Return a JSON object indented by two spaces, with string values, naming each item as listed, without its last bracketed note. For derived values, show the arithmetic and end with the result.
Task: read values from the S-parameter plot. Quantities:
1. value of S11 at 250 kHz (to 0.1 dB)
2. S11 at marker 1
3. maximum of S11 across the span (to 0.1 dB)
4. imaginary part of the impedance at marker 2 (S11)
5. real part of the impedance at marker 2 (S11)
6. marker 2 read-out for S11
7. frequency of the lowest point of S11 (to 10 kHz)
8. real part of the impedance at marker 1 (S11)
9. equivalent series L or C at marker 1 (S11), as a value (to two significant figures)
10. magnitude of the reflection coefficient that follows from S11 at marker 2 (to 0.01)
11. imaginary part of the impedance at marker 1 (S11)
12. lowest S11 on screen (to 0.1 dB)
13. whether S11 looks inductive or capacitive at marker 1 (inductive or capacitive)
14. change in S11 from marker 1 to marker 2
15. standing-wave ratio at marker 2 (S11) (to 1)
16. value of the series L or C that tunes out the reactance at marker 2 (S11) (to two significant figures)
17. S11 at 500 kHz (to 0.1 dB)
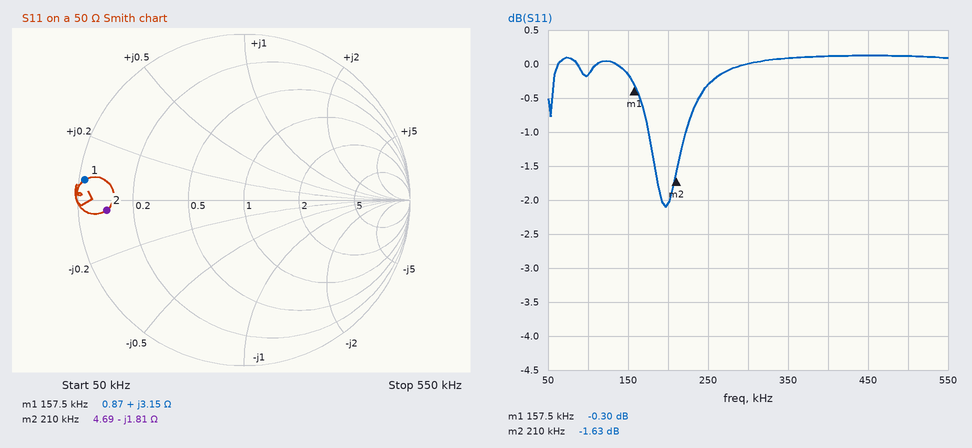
{
  "value of S11 at 250 kHz": "-0.3 dB",
  "S11 at marker 1": "-0.30 dB",
  "maximum of S11 across the span": "0.1 dB",
  "imaginary part of the impedance at marker 2": "-1.81 Ω",
  "real part of the impedance at marker 2": "4.69 Ω",
  "marker 2 read-out for S11": "-1.63 dB",
  "frequency of the lowest point of S11": "200 kHz",
  "real part of the impedance at marker 1": "0.87 Ω",
  "equivalent series L or C at marker 1 (S11), as a value": "L = 3.15 Ω/(2π × 157.5 kHz) ≈ 3.2 µH",
  "magnitude of the reflection coefficient that follows from S11 at marker 2": "10^(-1.63/20) ≈ 0.83",
  "imaginary part of the impedance at marker 1": "+3.15 Ω",
  "lowest S11 on screen": "-2.1 dB",
  "whether S11 looks inductive or capacitive at marker 1": "inductive",
  "change in S11 from marker 1 to marker 2": "-1.63 − (-0.3) = -1.33 dB",
  "standing-wave ratio at marker 2 (S11)": "11",
  "value of the series L or C that tunes out the reactance at marker 2 (S11)": "L = 1.81 Ω/(2π × 210 kHz) ≈ 1.4 µH",
  "S11 at 500 kHz": "0.1 dB"
}
